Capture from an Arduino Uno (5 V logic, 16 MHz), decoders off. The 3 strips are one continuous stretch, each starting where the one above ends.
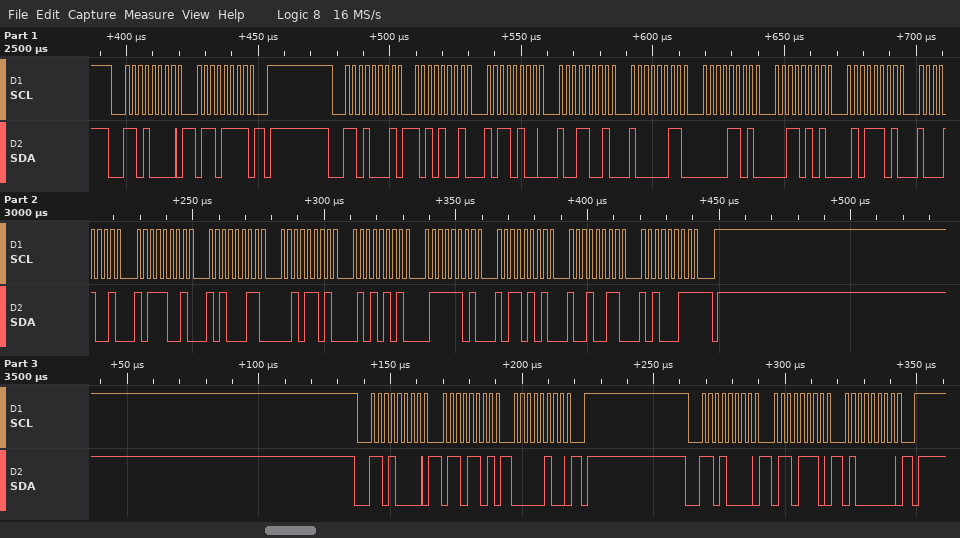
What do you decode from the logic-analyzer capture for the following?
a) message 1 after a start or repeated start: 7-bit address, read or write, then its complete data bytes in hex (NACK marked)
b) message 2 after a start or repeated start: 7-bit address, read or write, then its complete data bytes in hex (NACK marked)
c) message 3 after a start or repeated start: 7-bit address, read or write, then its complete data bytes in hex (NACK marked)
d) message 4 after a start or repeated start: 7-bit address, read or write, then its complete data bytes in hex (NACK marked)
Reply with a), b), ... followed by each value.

a) 0x68 write: 6F
b) 0x68 read: A9 B4 99 83 0D 35 5D 89 B9 A3 2D 55 7D B5 93 A3 NACK
c) 0x68 write: 6D 04
d) 0x68 write: 6E 40
